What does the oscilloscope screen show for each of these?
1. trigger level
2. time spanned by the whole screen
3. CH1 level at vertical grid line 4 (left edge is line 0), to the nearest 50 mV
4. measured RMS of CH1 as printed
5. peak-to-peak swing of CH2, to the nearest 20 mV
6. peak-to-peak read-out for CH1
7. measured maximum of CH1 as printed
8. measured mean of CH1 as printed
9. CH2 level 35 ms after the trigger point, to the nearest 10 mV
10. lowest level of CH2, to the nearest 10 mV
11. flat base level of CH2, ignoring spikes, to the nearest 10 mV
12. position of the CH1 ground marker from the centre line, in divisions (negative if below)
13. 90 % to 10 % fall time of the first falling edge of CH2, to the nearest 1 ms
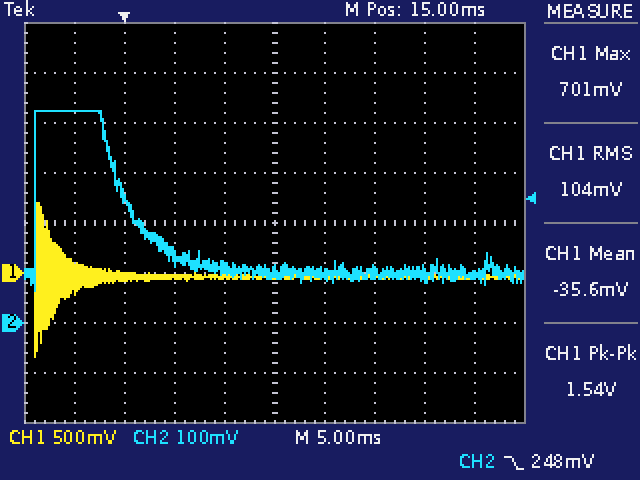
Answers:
248 mV
50 ms
-50 mV
104 mV
360 mV
1.54 V
701 mV
-35.6 mV
100 mV
60 mV
100 mV
-1.0 div
7 ms
